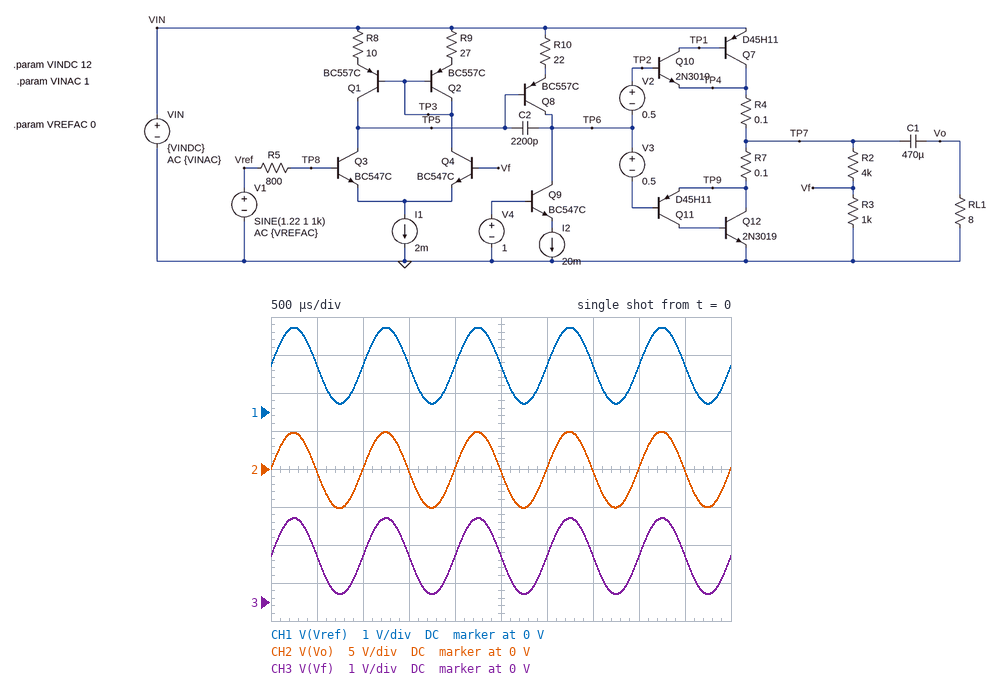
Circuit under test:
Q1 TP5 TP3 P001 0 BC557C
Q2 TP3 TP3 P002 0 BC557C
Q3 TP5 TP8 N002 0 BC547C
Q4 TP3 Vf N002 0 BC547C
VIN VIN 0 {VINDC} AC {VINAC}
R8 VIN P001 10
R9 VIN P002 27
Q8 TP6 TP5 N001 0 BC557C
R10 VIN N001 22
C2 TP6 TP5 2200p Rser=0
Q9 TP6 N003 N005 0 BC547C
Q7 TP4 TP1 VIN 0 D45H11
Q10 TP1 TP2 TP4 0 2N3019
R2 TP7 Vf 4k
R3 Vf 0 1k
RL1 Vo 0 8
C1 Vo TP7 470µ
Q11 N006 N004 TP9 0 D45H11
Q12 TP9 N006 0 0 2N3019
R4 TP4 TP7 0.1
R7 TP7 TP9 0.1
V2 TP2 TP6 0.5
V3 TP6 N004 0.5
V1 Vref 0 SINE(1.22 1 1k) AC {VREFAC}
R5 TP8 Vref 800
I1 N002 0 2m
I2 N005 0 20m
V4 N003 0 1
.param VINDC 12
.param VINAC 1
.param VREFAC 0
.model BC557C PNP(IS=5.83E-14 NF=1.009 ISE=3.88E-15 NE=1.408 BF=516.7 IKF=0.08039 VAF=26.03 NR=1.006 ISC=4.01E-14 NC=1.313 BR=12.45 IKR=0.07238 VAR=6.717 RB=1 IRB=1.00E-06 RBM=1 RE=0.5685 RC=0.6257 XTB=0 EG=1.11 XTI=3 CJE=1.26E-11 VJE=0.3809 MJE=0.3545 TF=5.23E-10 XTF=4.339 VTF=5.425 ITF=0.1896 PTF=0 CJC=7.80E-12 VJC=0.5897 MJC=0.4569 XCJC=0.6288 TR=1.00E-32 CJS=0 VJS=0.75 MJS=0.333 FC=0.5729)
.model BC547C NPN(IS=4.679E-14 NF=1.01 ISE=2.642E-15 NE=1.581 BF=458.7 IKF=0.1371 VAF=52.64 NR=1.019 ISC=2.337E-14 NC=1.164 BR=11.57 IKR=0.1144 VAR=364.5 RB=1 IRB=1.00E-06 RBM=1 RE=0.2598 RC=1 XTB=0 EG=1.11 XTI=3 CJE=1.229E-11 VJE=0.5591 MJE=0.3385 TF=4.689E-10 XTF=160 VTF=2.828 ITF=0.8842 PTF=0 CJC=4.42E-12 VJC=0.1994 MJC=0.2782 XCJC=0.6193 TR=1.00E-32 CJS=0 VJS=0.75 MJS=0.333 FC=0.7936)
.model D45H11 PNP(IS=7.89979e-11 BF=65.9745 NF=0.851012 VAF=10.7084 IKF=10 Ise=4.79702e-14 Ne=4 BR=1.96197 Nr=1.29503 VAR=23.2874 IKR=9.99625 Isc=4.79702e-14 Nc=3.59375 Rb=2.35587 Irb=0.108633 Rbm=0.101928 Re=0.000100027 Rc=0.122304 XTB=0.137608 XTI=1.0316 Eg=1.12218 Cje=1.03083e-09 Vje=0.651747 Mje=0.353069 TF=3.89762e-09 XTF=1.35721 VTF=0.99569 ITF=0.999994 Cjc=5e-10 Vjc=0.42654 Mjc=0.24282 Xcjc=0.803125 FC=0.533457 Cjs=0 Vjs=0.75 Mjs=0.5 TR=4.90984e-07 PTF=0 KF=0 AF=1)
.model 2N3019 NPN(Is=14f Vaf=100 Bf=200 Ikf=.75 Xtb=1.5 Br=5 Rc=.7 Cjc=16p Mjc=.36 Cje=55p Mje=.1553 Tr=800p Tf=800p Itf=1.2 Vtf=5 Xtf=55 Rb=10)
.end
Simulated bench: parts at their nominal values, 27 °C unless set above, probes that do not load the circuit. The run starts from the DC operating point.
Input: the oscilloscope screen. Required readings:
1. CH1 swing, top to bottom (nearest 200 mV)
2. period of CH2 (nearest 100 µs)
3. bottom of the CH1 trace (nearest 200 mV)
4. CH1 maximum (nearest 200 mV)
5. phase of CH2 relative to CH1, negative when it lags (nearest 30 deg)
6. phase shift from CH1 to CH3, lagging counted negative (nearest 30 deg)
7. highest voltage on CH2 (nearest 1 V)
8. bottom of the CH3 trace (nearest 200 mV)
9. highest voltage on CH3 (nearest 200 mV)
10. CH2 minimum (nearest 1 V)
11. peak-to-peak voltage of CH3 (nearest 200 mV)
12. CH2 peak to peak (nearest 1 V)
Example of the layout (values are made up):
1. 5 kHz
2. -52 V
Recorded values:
1. 2.0 V
2. 1.0 ms
3. 200 mV
4. 2.2 V
5. 0 deg
6. 0 deg
7. 5 V
8. 200 mV
9. 2.2 V
10. -5 V
11. 2.0 V
12. 10 V
